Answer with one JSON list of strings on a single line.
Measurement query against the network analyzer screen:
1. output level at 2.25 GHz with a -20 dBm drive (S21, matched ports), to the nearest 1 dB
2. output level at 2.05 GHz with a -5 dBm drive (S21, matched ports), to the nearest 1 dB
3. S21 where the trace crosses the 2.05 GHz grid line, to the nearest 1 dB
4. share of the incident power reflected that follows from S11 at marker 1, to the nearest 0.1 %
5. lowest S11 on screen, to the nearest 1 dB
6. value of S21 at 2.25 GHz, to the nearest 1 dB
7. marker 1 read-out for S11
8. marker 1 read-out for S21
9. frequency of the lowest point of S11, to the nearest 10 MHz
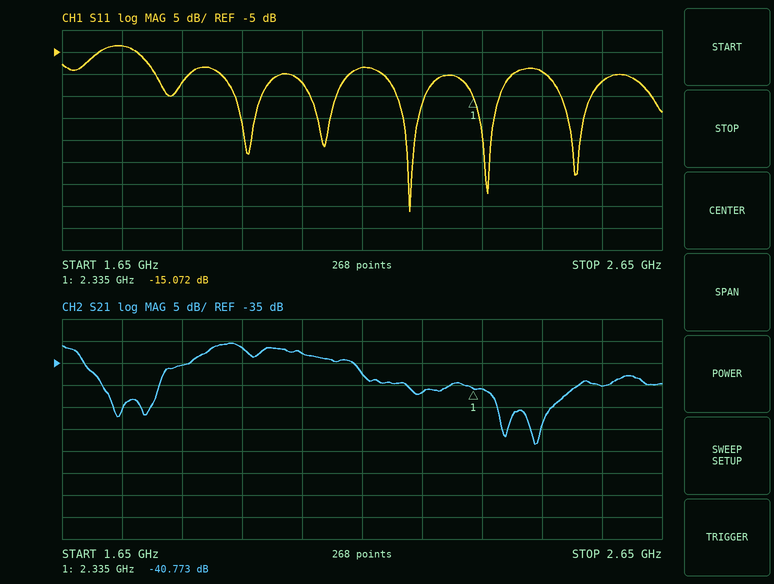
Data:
["-62 dBm", "-38 dBm", "-33 dB", "3.1 %", "-41 dB", "-42 dB", "-15.072 dB", "-40.773 dB", "2.23 GHz"]
